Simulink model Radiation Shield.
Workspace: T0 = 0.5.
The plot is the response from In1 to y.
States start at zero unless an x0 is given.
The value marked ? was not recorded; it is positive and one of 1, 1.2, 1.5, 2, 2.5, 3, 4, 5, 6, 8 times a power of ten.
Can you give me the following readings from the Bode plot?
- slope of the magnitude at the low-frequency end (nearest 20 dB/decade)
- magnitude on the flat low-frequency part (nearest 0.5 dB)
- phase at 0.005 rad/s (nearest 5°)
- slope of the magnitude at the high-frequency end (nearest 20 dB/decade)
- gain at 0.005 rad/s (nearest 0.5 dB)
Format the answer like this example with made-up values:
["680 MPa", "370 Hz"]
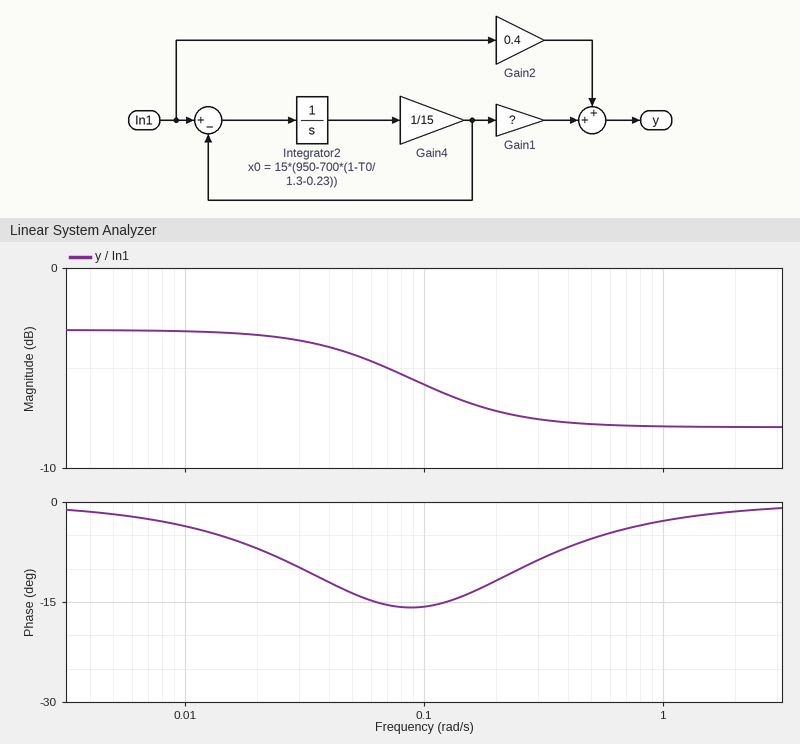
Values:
["0 dB/decade", "-3.0 dB", "0°", "0 dB/decade", "-3.0 dB"]
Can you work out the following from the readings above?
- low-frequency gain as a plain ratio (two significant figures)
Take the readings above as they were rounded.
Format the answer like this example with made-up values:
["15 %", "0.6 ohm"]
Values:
["0.71"]
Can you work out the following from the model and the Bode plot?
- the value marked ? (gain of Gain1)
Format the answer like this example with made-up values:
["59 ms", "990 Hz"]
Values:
["0.3"]
